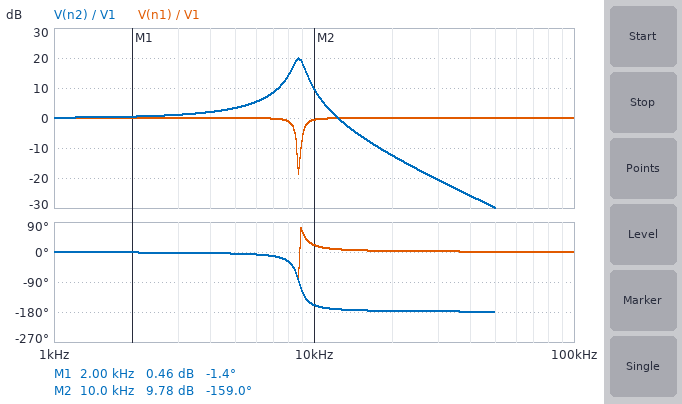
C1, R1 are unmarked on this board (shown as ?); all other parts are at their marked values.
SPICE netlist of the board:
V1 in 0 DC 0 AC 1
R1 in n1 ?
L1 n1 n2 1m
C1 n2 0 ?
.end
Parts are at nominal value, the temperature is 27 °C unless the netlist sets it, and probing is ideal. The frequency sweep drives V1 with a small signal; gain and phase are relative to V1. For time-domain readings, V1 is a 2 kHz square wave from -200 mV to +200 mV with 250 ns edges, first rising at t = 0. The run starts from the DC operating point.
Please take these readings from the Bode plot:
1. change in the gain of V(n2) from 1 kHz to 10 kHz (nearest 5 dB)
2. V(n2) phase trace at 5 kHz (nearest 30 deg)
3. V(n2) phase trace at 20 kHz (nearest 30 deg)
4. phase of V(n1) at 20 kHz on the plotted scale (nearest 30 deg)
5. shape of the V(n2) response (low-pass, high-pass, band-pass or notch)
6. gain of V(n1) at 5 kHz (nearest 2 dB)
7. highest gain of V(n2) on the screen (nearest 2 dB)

10 dB
0 deg
-180 deg
0 deg
band-pass
0 dB
20 dB
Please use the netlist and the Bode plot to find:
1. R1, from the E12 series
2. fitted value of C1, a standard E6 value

5.6 Ω
330 nF
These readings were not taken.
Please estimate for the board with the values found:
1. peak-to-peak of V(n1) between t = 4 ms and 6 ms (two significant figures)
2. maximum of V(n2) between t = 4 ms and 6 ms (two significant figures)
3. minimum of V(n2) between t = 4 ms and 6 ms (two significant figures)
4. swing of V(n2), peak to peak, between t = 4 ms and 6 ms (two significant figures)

450 mV
460 mV
-460 mV
920 mV
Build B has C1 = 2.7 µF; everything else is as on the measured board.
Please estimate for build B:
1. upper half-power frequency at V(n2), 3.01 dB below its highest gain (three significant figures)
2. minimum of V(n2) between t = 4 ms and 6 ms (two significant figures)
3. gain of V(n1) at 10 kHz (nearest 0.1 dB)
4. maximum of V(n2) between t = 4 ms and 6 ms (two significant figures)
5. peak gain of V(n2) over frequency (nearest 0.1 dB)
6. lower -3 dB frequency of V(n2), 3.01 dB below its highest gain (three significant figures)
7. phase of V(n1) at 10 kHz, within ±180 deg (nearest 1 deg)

3.42 kHz
-440 mV
0 dB
440 mV
10.8 dB
2.51 kHz
6 deg
